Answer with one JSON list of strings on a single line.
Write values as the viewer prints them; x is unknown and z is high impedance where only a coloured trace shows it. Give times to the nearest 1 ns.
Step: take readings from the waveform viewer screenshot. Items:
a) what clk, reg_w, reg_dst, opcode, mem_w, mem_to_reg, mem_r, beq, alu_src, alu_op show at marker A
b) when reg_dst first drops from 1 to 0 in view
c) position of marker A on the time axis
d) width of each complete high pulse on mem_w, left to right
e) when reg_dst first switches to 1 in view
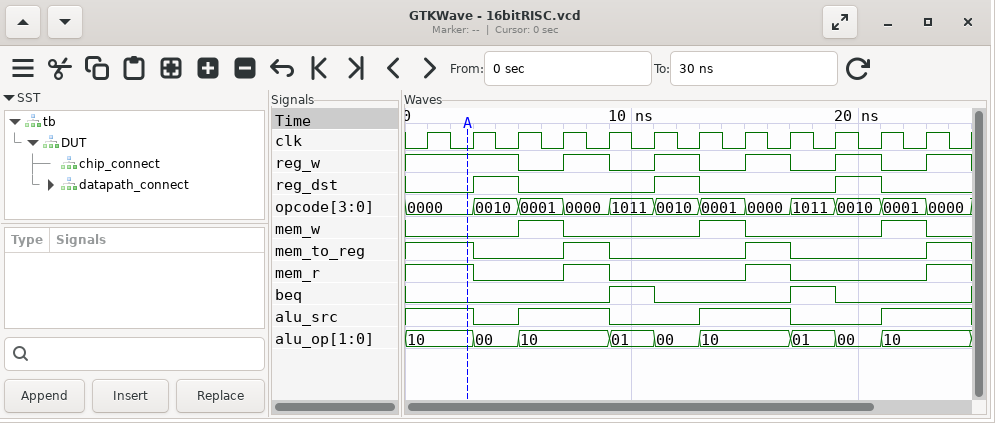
["clk=0, reg_w=1, reg_dst=0, opcode=0000, mem_w=0, mem_to_reg=1, mem_r=1, beq=0, alu_src=1, alu_op=10", "5 ns", "3 ns", "2 ns, 2 ns, 2 ns", "3 ns"]
